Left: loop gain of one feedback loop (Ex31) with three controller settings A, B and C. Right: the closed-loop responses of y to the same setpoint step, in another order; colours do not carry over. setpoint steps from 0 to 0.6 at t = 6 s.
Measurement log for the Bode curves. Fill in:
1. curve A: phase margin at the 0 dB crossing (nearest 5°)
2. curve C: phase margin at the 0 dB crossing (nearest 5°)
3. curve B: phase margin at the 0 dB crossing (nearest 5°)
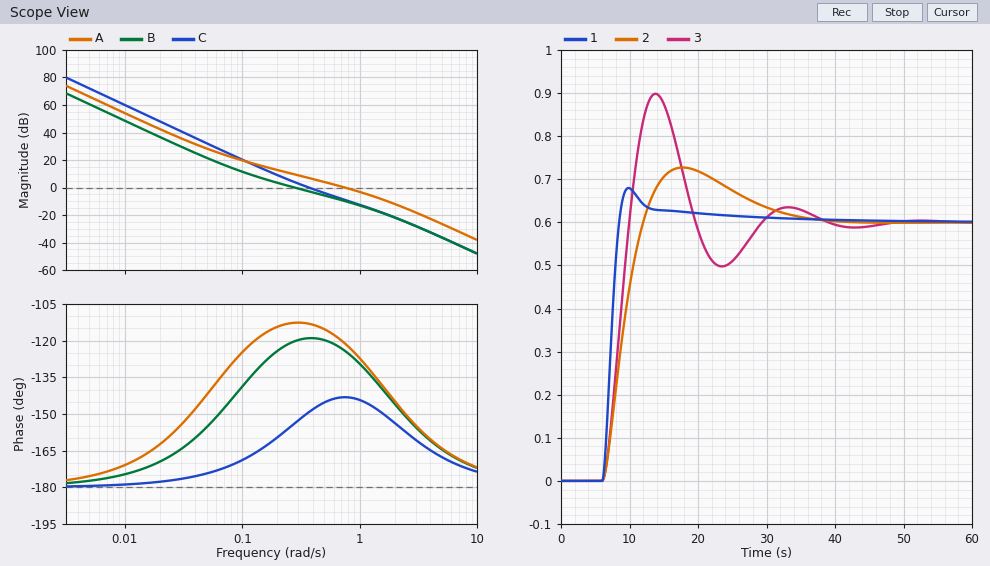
60°
30°
60°
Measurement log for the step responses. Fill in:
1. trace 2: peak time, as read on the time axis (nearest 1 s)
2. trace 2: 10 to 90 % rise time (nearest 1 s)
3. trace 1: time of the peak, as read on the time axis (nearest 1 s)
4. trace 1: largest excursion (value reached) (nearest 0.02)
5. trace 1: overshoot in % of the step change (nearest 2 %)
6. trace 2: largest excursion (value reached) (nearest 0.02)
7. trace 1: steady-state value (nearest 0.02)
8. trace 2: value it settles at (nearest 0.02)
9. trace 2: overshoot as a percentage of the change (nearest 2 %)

18 s
4 s
10 s
0.68
14 %
0.72
0.60
0.60
22 %
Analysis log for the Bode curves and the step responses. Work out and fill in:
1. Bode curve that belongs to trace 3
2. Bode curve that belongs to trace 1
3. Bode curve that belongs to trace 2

C
A
B
